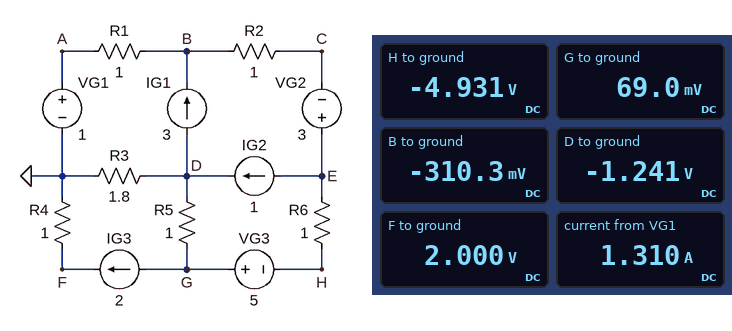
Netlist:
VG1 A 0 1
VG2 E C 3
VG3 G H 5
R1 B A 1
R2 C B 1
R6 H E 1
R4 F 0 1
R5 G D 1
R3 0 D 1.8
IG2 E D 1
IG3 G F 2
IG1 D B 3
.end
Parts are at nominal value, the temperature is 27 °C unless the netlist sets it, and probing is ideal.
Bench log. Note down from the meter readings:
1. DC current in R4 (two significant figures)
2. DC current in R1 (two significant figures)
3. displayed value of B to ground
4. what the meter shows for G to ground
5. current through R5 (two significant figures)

2.0 A
1.3 A
-310.3 mV
69.0 mV
1.3 A
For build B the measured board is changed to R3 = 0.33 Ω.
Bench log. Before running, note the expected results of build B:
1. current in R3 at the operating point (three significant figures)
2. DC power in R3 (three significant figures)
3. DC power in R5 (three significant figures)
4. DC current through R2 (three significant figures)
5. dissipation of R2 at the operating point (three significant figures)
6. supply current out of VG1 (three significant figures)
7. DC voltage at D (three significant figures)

924 mA
282 mW
1.16 W
4.08 A
16.6 W
1.08 A
-305 mV
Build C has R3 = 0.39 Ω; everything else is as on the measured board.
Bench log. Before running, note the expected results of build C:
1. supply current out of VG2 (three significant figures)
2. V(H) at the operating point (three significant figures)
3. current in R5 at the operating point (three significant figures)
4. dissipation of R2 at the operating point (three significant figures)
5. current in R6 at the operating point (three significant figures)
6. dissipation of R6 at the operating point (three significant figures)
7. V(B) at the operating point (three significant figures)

4.09 A
-4.27 V
1.09 A
16.7 W
3.09 A
9.54 W
-88.8 mV
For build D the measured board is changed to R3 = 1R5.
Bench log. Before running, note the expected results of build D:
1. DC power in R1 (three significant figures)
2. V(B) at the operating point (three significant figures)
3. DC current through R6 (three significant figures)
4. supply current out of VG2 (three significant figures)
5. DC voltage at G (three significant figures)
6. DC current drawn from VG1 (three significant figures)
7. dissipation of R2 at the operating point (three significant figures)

1.62 W
-273 mV
3.27 A
4.27 A
182 mV
1.27 A
18.3 W
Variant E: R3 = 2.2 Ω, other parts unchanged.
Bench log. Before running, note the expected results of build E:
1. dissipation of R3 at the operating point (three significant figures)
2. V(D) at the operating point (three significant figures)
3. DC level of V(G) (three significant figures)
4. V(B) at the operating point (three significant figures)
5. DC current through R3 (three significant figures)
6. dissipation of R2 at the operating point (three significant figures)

916 mW
-1.42 V
-64.5 mV
-355 mV
645 mA
19.0 W
